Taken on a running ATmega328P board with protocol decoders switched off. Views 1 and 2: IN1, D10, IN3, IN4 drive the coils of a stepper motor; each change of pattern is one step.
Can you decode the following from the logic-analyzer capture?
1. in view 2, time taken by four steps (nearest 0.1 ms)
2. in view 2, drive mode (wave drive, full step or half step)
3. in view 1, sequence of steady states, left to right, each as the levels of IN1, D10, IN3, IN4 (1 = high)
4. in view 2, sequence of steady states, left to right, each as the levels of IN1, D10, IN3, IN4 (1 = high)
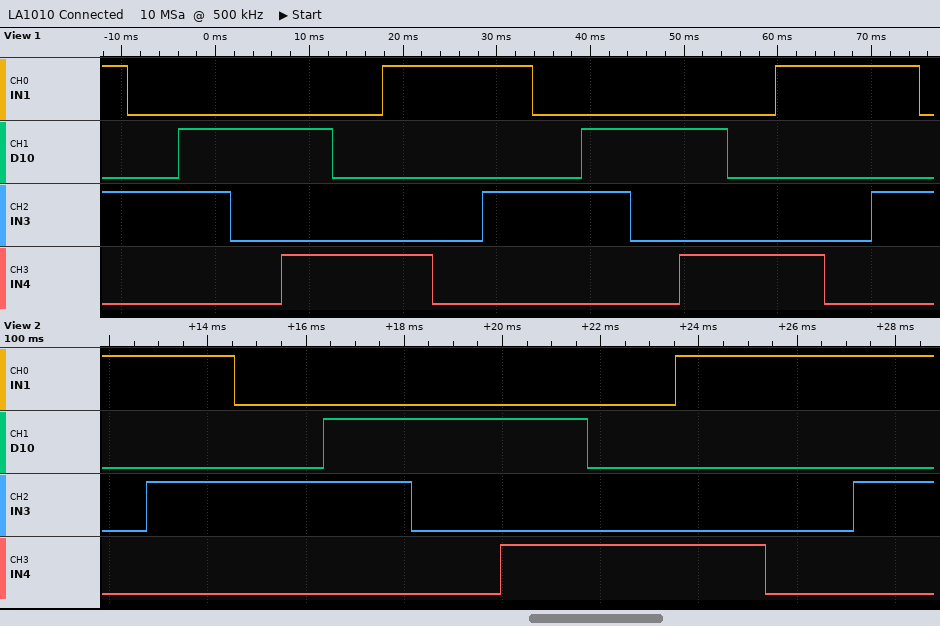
7.2 ms
half step
1010 0010 0110 0100 0101 0001 1001 1000 1010 0010 0110 0100 0101 0001 1001 1000 1010 0010
1000 1010 0010 0110 0100 0101 0001 1001 1000 1010
